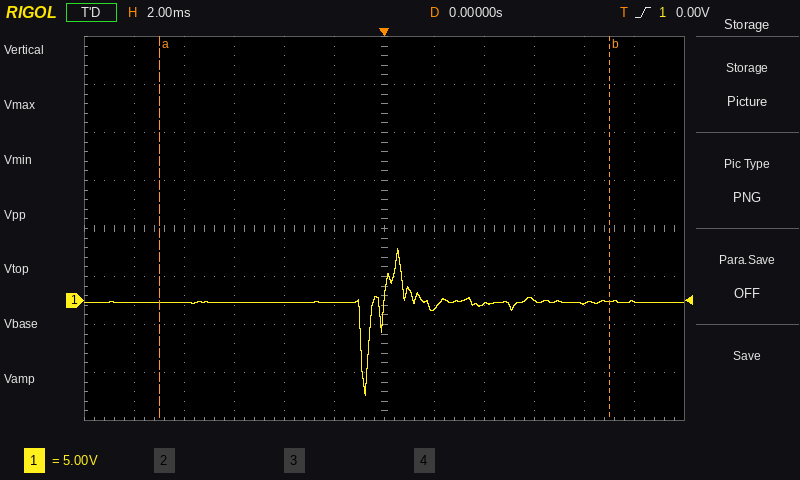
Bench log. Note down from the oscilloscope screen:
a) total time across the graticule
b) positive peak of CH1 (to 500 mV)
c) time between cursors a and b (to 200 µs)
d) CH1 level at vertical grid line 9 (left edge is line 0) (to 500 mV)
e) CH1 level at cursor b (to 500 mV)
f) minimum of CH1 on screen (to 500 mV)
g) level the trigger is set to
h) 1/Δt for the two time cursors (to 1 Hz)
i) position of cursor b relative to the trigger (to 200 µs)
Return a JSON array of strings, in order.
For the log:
["24 ms", "5.5 V", "18.0 ms", "0.0 V", "0.0 V", "-10.0 V", "0.00 V", "56 Hz", "+9.0 ms"]
